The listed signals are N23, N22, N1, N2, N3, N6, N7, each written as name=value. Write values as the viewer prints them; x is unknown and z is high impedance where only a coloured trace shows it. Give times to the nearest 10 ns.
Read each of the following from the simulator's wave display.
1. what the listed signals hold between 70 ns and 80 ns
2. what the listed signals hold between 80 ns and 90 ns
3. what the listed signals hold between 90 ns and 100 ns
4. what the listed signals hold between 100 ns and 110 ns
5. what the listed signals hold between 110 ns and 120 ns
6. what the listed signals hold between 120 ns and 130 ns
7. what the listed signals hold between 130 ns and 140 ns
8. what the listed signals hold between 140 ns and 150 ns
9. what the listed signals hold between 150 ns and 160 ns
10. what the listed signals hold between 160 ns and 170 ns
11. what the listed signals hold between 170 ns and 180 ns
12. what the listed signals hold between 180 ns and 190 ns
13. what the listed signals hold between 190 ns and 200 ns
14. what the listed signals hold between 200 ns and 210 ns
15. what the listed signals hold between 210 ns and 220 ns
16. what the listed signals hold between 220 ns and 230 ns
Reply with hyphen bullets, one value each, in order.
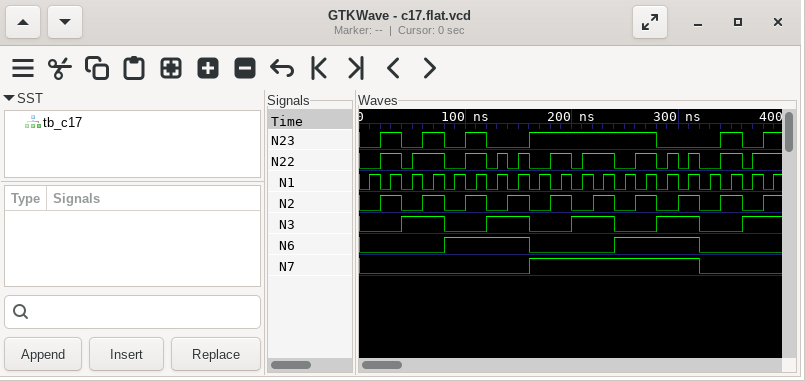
- N23=1, N22=1, N1=1, N2=1, N3=1, N6=0, N7=0
- N23=0, N22=0, N1=0, N2=0, N3=0, N6=1, N7=0
- N23=0, N22=0, N1=1, N2=0, N3=0, N6=1, N7=0
- N23=1, N22=1, N1=0, N2=1, N3=0, N6=1, N7=0
- N23=1, N22=1, N1=1, N2=1, N3=0, N6=1, N7=0
- N23=0, N22=0, N1=0, N2=0, N3=1, N6=1, N7=0
- N23=0, N22=1, N1=1, N2=0, N3=1, N6=1, N7=0
- N23=0, N22=0, N1=0, N2=1, N3=1, N6=1, N7=0
- N23=0, N22=1, N1=1, N2=1, N3=1, N6=1, N7=0
- N23=1, N22=0, N1=0, N2=0, N3=0, N6=0, N7=1
- N23=1, N22=0, N1=1, N2=0, N3=0, N6=0, N7=1
- N23=1, N22=1, N1=0, N2=1, N3=0, N6=0, N7=1
- N23=1, N22=1, N1=1, N2=1, N3=0, N6=0, N7=1
- N23=1, N22=0, N1=0, N2=0, N3=1, N6=0, N7=1
- N23=1, N22=1, N1=1, N2=0, N3=1, N6=0, N7=1
- N23=1, N22=1, N1=0, N2=1, N3=1, N6=0, N7=1
